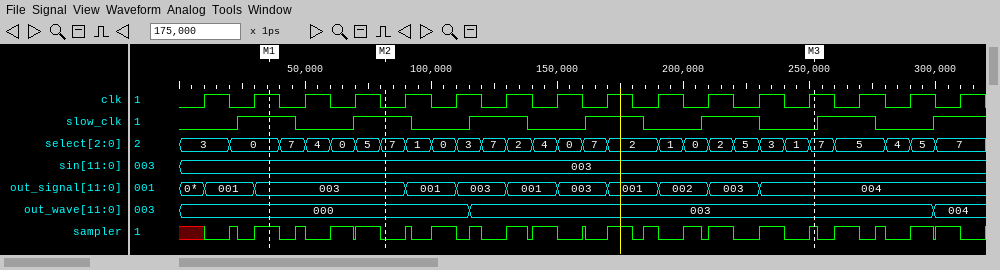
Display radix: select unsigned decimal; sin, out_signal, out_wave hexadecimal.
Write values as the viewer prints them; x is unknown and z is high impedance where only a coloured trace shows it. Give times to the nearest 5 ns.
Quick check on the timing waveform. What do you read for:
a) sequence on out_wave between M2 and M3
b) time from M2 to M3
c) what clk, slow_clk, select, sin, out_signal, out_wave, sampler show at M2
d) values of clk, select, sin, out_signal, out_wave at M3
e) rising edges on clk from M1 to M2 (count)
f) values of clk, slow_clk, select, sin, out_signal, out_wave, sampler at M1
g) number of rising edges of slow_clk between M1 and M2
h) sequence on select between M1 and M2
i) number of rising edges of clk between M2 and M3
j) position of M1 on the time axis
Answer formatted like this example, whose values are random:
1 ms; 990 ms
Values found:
000, 003; 170 ns; clk=0, slow_clk=1, select=7, sin=003, out_signal=003, out_wave=000, sampler=0; clk=1, select=7, sin=003, out_signal=004, out_wave=003; 2; clk=1, slow_clk=1, select=0, sin=003, out_signal=003, out_wave=000, sampler=1; 1; 0, 7, 4, 0, 5, 7; 9; 35 ns
